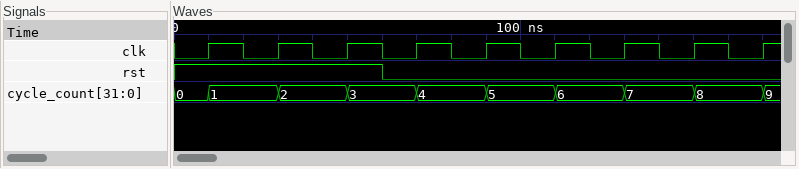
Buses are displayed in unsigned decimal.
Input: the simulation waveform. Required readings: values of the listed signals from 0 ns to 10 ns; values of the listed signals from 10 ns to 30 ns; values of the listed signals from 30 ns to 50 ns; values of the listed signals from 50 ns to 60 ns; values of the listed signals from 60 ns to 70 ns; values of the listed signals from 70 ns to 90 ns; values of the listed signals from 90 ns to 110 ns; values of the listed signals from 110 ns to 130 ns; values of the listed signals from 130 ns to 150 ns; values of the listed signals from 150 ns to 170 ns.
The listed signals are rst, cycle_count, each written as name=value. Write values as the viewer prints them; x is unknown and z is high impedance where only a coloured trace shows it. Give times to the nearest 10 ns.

rst=1, cycle_count=0
rst=1, cycle_count=1
rst=1, cycle_count=2
rst=1, cycle_count=3
rst=0, cycle_count=3
rst=0, cycle_count=4
rst=0, cycle_count=5
rst=0, cycle_count=6
rst=0, cycle_count=7
rst=0, cycle_count=8
